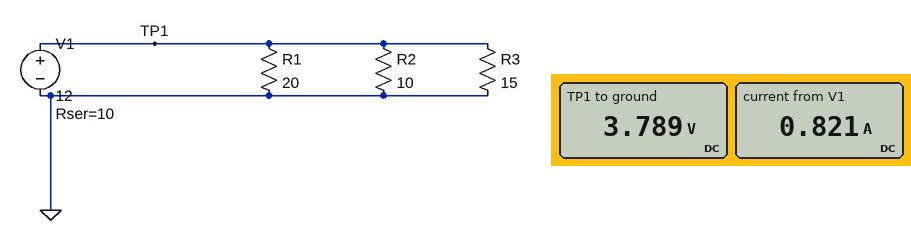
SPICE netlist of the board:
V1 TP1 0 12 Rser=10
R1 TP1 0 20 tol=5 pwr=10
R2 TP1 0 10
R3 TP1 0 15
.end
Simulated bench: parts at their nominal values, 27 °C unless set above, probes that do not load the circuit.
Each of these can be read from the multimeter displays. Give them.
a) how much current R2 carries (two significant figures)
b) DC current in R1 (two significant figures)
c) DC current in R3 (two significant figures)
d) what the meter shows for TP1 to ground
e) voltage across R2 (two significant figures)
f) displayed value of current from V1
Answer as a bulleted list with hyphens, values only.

- 380 mA
- 190 mA
- 250 mA
- 3.789 V
- 3.8 V
- 0.821 A
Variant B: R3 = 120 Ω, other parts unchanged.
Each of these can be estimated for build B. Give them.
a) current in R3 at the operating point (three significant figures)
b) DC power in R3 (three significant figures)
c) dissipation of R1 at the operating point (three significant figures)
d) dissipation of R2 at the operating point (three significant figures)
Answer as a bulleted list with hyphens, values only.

- 38.7 mA
- 180 mW
- 1.08 W
- 2.16 W
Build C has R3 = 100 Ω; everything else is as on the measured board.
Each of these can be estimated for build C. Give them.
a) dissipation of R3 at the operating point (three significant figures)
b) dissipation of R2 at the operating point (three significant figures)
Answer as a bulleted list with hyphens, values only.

- 213 mW
- 2.13 W
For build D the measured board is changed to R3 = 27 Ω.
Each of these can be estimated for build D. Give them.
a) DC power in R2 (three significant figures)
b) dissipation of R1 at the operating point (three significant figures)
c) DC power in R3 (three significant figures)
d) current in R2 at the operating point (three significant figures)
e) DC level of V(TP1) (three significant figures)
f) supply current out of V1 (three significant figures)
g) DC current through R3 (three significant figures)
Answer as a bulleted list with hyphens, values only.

- 1.75 W
- 874 mW
- 647 mW
- 418 mA
- 4.18 V
- 782 mA
- 155 mA
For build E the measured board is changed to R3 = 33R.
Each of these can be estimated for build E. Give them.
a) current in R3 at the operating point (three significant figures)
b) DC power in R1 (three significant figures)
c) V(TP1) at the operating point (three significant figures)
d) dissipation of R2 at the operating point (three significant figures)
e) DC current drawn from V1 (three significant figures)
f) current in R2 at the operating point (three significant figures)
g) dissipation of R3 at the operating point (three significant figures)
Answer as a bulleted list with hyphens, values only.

- 130 mA
- 916 mW
- 4.28 V
- 1.83 W
- 772 mA
- 428 mA
- 555 mW
